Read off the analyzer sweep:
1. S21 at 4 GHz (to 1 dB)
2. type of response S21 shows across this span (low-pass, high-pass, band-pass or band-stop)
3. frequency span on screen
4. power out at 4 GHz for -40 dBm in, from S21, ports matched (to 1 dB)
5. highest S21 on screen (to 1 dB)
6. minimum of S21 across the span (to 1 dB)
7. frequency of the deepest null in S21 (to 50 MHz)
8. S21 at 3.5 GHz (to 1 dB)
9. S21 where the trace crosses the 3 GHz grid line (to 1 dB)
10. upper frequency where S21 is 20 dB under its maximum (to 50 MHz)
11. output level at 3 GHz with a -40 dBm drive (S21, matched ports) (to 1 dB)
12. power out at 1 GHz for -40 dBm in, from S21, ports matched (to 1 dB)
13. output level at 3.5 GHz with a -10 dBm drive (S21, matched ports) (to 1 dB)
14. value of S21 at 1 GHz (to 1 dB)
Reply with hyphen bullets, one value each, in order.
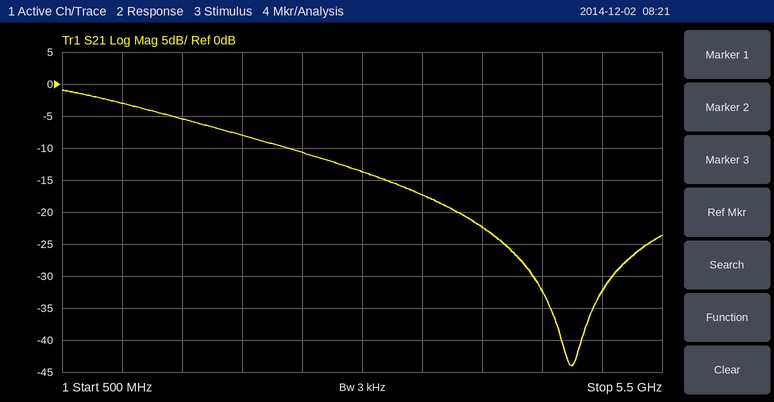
- -22 dB
- low-pass
- 5 GHz
- -62 dBm
- -1 dB
- -44 dB
- 4.75 GHz
- -17 dB
- -14 dB
- 3.90 GHz
- -54 dBm
- -43 dBm
- -27 dBm
- -3 dB
